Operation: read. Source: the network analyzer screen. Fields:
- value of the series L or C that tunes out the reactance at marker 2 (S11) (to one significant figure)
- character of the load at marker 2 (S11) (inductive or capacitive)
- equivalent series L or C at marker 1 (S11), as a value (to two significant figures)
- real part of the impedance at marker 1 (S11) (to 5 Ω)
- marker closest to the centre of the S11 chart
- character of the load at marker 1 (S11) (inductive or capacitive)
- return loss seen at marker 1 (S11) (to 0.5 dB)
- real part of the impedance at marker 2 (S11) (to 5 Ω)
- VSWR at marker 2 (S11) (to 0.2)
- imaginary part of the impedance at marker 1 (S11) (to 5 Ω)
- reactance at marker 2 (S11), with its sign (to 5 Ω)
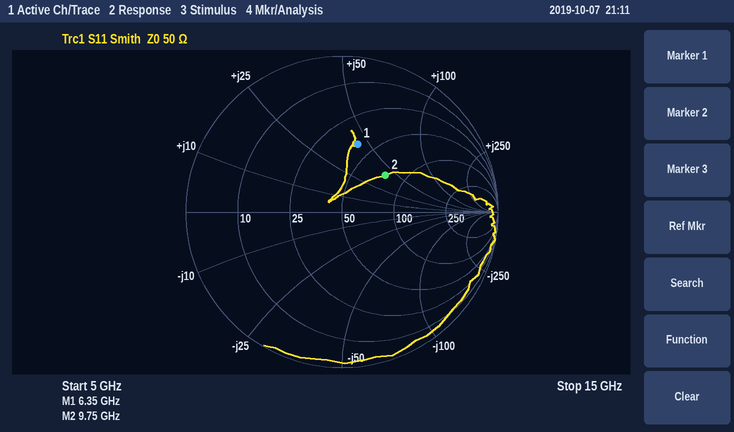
400 fF
inductive
1.1 nH
40 Ω
marker 2
inductive
7.0 dB
75 Ω
2.2
+45 Ω
+40 Ω
